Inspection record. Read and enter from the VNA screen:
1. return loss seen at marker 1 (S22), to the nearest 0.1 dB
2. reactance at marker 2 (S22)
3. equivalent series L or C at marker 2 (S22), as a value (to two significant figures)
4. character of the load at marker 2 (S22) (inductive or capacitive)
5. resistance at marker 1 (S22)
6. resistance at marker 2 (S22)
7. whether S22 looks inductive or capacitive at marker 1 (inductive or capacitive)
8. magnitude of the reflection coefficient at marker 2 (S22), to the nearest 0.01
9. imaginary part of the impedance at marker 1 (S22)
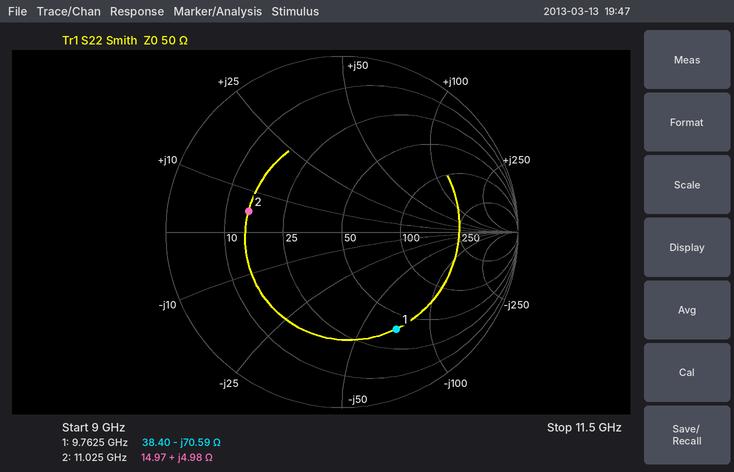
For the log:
4.0 dB
+4.98 Ω
72 pH
inductive
38.40 Ω
14.97 Ω
capacitive
0.54
-70.59 Ω
